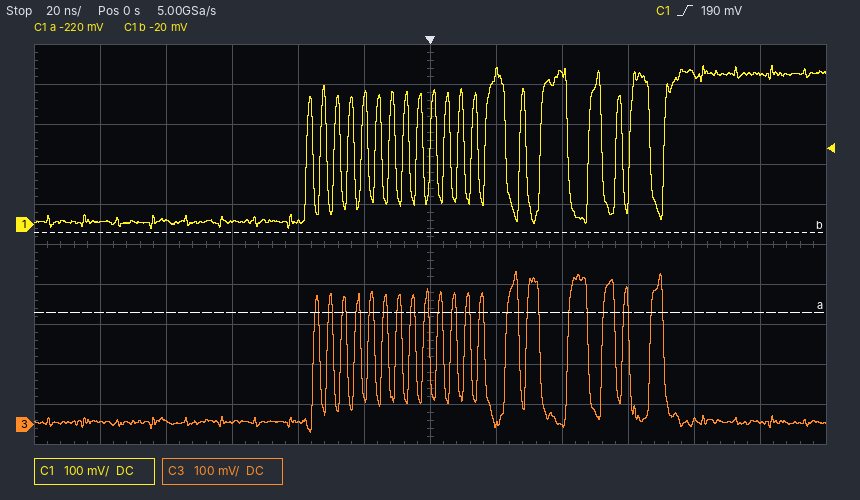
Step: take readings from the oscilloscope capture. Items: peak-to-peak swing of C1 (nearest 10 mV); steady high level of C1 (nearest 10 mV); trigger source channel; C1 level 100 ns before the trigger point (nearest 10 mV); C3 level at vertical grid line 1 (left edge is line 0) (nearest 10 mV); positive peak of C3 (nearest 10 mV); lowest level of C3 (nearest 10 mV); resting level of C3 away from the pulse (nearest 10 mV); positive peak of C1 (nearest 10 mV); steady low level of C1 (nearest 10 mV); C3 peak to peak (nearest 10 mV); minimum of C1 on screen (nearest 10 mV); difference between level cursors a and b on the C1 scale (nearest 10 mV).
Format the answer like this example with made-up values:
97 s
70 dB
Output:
410 mV
380 mV
C1
10 mV
10 mV
380 mV
-20 mV
10 mV
400 mV
10 mV
400 mV
-10 mV
200 mV
